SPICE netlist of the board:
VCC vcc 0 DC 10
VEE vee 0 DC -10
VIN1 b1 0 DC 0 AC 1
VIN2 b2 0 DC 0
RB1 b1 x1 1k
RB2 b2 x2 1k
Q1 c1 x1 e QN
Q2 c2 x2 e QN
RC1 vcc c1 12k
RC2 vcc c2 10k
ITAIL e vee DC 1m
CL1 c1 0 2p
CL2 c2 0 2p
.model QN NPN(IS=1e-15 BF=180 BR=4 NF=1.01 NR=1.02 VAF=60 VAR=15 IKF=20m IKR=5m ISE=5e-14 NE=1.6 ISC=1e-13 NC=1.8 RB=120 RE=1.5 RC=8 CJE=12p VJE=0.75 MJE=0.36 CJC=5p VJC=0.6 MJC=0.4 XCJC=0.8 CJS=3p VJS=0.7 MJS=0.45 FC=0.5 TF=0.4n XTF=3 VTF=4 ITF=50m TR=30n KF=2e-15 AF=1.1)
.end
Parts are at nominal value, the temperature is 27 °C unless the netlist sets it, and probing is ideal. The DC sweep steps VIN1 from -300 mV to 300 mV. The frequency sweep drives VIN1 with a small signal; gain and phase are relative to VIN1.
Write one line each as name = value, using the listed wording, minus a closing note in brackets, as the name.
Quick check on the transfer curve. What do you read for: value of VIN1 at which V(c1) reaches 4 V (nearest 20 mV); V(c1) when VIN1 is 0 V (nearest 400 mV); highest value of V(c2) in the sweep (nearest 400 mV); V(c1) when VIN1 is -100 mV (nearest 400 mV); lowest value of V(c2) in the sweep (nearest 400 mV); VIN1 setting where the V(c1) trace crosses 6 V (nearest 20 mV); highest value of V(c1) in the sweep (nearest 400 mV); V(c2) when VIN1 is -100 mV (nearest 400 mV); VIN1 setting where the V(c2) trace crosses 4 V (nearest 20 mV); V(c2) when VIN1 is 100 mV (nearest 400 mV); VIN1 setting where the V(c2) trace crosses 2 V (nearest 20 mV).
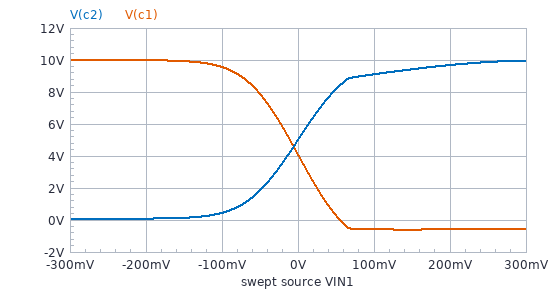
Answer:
value of VIN1 at which V(c1) reaches 4 V = 0 V
V(c1) when VIN1 is 0 V = 4.0 V
highest value of V(c2) in the sweep = 10.0 V
V(c1) when VIN1 is -100 mV = 9.6 V
lowest value of V(c2) in the sweep = 0 V
VIN1 setting where the V(c1) trace crosses 6 V = -20 mV
highest value of V(c1) in the sweep = 10.0 V
V(c2) when VIN1 is -100 mV = 400 mV
VIN1 setting where the V(c2) trace crosses 4 V = -20 mV
V(c2) when VIN1 is 100 mV = 9.2 V
VIN1 setting where the V(c2) trace crosses 2 V = -40 mV
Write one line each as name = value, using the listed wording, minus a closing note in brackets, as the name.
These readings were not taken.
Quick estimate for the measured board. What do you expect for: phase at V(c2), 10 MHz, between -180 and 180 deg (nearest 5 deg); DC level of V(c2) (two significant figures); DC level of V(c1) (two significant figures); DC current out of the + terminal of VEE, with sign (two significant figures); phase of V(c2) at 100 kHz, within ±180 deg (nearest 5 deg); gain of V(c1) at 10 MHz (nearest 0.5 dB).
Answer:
phase at V(c2), 10 MHz, between -180 and 180 deg = -95 deg
DC level of V(c2) = 5.0 V
DC level of V(c1) = 4.1 V
DC current out of the + terminal of VEE, with sign = -1.0 mA
phase of V(c2) at 100 kHz, within ±180 deg = -15 deg
gain of V(c1) at 10 MHz = 9.0 dB
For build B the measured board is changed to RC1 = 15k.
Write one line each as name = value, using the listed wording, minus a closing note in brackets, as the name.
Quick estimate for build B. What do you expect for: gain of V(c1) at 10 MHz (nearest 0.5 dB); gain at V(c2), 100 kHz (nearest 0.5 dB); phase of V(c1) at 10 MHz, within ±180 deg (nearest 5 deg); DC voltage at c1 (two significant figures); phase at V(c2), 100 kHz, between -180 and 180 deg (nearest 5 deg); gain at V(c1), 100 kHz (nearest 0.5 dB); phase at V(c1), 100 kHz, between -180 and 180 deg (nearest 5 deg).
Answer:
gain of V(c1) at 10 MHz = 8.0 dB
gain at V(c2), 100 kHz = 36.5 dB
phase of V(c1) at 10 MHz, within ±180 deg = 70 deg
DC voltage at c1 = 2.7 V
phase at V(c2), 100 kHz, between -180 and 180 deg = -20 deg
gain at V(c1), 100 kHz = 40.0 dB
phase at V(c1), 100 kHz, between -180 and 180 deg = 160 deg
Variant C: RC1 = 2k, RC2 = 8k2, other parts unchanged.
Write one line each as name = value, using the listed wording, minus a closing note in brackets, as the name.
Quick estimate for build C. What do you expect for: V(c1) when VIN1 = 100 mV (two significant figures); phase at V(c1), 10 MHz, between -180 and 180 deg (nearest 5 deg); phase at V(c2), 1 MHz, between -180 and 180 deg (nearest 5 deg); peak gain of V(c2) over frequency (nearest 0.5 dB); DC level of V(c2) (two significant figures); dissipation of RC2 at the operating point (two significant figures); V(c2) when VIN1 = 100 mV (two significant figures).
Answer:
V(c1) when VIN1 = 100 mV = 8.1 V
phase at V(c1), 10 MHz, between -180 and 180 deg = 105 deg
phase at V(c2), 1 MHz, between -180 and 180 deg = -55 deg
peak gain of V(c2) over frequency = 36.0 dB
DC level of V(c2) = 6.0 V
dissipation of RC2 at the operating point = 1.9 mW
V(c2) when VIN1 = 100 mV = 9.7 V
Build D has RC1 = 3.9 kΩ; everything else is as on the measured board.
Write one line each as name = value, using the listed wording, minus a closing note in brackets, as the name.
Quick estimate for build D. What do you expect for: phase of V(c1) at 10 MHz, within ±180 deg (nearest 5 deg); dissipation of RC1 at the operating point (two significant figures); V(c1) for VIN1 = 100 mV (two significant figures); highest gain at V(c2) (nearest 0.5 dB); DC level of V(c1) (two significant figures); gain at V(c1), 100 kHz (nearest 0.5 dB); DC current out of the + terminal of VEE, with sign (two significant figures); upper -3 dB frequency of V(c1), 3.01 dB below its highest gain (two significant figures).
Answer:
phase of V(c1) at 10 MHz, within ±180 deg = 90 deg
dissipation of RC1 at the operating point = 1.0 mW
V(c1) for VIN1 = 100 mV = 6.3 V
highest gain at V(c2) = 37.5 dB
DC level of V(c1) = 8.0 V
gain at V(c1), 100 kHz = 29.0 dB
DC current out of the + terminal of VEE, with sign = -1.0 mA
upper -3 dB frequency of V(c1), 3.01 dB below its highest gain = 570 kHz
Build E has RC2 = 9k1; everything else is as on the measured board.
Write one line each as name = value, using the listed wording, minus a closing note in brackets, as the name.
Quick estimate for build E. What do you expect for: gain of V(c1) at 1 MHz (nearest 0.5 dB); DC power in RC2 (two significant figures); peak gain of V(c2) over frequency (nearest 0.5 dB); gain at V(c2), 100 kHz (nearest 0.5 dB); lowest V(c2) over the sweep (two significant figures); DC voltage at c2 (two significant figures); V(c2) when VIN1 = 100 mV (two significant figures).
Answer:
gain of V(c1) at 1 MHz = 29.5 dB
DC power in RC2 = 2.3 mW
peak gain of V(c2) over frequency = 36.5 dB
gain at V(c2), 100 kHz = 36.0 dB
lowest V(c2) over the sweep = 970 mV
DC voltage at c2 = 5.4 V
V(c2) when VIN1 = 100 mV = 9.2 V
